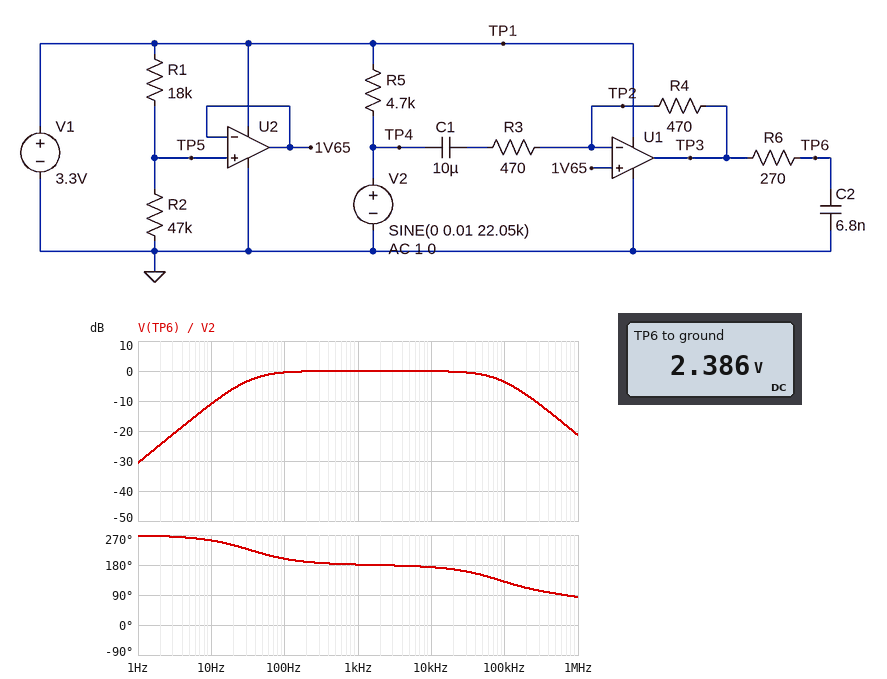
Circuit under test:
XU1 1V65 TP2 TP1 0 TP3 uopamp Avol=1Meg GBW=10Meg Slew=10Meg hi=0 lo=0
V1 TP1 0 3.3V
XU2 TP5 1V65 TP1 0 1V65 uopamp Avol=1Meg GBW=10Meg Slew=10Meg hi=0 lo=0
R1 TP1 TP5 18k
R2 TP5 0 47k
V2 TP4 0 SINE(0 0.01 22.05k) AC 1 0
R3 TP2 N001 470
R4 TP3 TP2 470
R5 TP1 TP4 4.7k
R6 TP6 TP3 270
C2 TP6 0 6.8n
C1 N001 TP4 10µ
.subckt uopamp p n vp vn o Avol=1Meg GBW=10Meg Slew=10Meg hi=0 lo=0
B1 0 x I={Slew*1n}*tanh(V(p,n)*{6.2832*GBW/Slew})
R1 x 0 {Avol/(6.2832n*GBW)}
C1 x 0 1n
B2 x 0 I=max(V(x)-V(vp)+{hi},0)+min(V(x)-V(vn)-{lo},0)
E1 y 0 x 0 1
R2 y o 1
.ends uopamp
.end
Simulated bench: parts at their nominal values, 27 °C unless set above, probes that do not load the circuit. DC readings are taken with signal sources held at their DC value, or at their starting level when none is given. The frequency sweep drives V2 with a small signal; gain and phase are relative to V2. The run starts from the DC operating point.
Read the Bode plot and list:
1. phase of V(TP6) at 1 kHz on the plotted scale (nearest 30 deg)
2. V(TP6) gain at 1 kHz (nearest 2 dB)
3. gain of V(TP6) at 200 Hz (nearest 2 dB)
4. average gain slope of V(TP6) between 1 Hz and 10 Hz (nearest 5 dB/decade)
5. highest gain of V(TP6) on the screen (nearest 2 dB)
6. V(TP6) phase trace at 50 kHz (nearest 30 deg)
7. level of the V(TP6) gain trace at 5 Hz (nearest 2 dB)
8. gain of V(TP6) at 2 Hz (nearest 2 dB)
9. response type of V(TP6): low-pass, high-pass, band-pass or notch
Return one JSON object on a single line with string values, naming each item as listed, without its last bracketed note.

{"phase of V(TP6) at 1 kHz on the plotted scale": "180 deg", "V(TP6) gain at 1 kHz": "0 dB", "gain of V(TP6) at 200 Hz": "0 dB", "average gain slope of V(TP6) between 1 Hz and 10 Hz": "20 dB/decade", "highest gain of V(TP6) on the screen": "0 dB", "V(TP6) phase trace at 50 kHz": "150 deg", "level of the V(TP6) gain trace at 5 Hz": "-16 dB", "gain of V(TP6) at 2 Hz": "-24 dB", "response type of V(TP6): low-pass, high-pass, band-pass or notch": "band-pass"}
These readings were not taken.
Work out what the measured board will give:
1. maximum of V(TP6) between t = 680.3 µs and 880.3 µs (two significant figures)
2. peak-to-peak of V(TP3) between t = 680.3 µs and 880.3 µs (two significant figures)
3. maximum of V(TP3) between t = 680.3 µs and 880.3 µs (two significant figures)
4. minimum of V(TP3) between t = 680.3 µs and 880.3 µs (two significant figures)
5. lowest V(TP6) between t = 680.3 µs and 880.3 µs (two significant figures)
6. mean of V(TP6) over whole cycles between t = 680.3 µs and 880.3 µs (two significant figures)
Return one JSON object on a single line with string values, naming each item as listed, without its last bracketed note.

{"maximum of V(TP6) between t = 680.3 µs and 880.3 µs": "2.4 V", "peak-to-peak of V(TP3) between t = 680.3 µs and 880.3 µs": "20 mV", "maximum of V(TP3) between t = 680.3 µs and 880.3 µs": "2.4 V", "minimum of V(TP3) between t = 680.3 µs and 880.3 µs": "2.4 V", "lowest V(TP6) between t = 680.3 µs and 880.3 µs": "2.4 V", "mean of V(TP6) over whole cycles between t = 680.3 µs and 880.3 µs": "2.4 V"}
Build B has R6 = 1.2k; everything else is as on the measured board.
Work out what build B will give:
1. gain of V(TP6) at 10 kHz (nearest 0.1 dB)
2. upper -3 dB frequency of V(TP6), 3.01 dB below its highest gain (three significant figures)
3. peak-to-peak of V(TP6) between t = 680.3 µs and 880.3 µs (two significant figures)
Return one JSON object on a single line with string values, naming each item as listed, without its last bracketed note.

{"gain of V(TP6) at 10 kHz": "-1.0 dB", "upper -3 dB frequency of V(TP6), 3.01 dB below its highest gain": "19.6 kHz", "peak-to-peak of V(TP6) between t = 680.3 µs and 880.3 µs": "13 mV"}
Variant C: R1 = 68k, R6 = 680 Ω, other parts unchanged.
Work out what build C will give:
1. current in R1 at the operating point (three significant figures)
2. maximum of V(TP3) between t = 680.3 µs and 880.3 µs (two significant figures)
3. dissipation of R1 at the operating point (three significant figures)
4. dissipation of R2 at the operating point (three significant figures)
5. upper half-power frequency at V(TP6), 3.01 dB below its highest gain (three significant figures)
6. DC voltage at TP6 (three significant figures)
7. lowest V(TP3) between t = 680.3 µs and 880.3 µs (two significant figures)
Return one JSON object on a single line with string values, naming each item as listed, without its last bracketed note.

{"current in R1 at the operating point": "28.7 µA", "maximum of V(TP3) between t = 680.3 µs and 880.3 µs": "1.4 V", "dissipation of R1 at the operating point": "56.0 µW", "dissipation of R2 at the operating point": "38.7 µW", "upper half-power frequency at V(TP6), 3.01 dB below its highest gain": "34.5 kHz", "DC voltage at TP6": "1.35 V", "lowest V(TP3) between t = 680.3 µs and 880.3 µs": "1.3 V"}
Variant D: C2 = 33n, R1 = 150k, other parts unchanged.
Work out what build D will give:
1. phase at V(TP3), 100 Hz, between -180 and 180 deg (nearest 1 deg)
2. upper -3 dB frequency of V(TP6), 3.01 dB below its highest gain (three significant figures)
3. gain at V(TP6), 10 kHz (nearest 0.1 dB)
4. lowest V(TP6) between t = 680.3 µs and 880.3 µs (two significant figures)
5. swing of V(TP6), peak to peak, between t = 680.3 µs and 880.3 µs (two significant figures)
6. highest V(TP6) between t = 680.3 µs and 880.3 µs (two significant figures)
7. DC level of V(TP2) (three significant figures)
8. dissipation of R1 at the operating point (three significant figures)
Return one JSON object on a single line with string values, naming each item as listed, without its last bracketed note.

{"phase at V(TP3), 100 Hz, between -180 and 180 deg": "-161 deg", "upper -3 dB frequency of V(TP6), 3.01 dB below its highest gain": "17.9 kHz", "gain at V(TP6), 10 kHz": "-1.2 dB", "lowest V(TP6) between t = 680.3 µs and 880.3 µs": "780 mV", "swing of V(TP6), peak to peak, between t = 680.3 µs and 880.3 µs": "13 mV", "highest V(TP6) between t = 680.3 µs and 880.3 µs": "790 mV", "DC level of V(TP2)": "787 mV", "dissipation of R1 at the operating point": "42.1 µW"}
